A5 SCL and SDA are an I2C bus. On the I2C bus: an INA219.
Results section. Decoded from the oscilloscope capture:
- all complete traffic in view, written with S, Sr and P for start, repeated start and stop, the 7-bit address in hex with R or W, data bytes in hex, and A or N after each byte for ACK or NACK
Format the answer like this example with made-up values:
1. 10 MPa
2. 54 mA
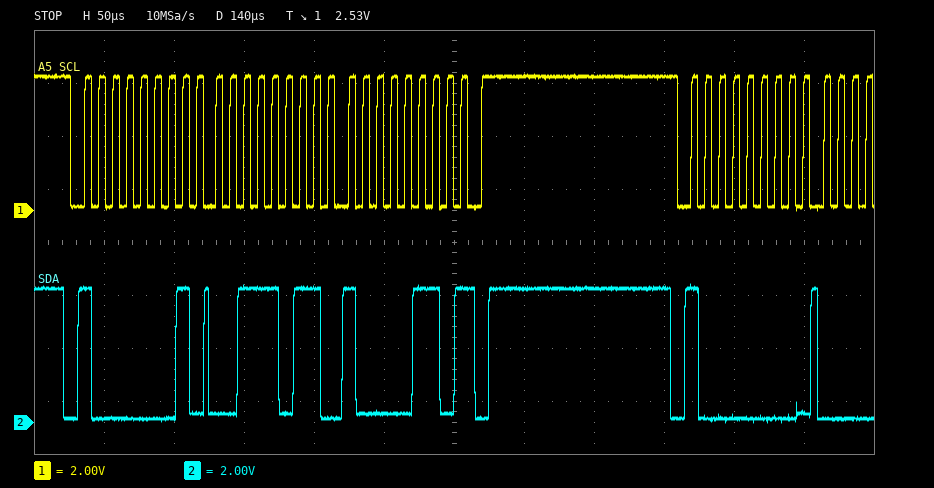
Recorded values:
1. S 40R A 3B A 86 N P S 40W A
